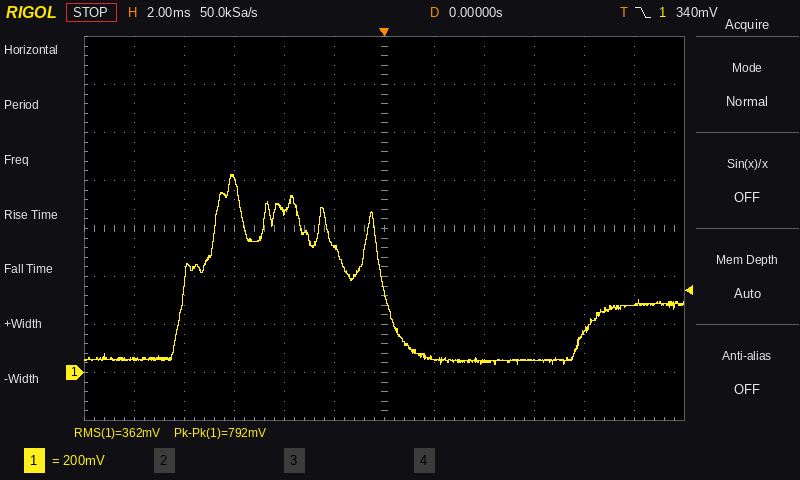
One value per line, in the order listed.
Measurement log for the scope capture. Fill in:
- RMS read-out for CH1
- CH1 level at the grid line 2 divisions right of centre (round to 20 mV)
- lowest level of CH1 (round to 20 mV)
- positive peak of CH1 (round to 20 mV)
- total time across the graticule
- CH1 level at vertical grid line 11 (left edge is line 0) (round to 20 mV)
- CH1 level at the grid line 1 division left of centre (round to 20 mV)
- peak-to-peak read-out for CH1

362 mV
40 mV
40 mV
820 mV
24 ms
280 mV
520 mV
792 mV
